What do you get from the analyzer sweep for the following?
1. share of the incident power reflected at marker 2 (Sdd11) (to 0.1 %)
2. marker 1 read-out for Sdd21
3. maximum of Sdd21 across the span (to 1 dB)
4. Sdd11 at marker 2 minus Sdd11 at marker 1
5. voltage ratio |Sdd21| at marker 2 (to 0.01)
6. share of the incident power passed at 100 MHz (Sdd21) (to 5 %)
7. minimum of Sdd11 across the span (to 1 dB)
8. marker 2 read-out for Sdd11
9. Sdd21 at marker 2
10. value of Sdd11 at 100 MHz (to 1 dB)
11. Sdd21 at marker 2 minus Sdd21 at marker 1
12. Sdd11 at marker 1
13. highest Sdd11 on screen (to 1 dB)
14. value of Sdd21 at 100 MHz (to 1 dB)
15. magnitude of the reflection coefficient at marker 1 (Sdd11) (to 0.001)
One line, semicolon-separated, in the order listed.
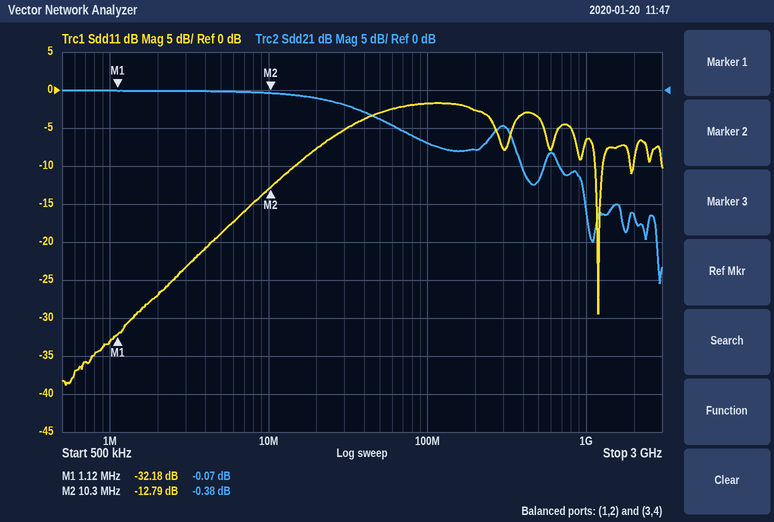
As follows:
5.3 %; -0.07 dB; 0 dB; 19.39 dB; 0.96; 20 %; -39 dB; -12.79 dB; -0.38 dB; -2 dB; -0.31 dB; -32.18 dB; -2 dB; -7 dB; 0.025
